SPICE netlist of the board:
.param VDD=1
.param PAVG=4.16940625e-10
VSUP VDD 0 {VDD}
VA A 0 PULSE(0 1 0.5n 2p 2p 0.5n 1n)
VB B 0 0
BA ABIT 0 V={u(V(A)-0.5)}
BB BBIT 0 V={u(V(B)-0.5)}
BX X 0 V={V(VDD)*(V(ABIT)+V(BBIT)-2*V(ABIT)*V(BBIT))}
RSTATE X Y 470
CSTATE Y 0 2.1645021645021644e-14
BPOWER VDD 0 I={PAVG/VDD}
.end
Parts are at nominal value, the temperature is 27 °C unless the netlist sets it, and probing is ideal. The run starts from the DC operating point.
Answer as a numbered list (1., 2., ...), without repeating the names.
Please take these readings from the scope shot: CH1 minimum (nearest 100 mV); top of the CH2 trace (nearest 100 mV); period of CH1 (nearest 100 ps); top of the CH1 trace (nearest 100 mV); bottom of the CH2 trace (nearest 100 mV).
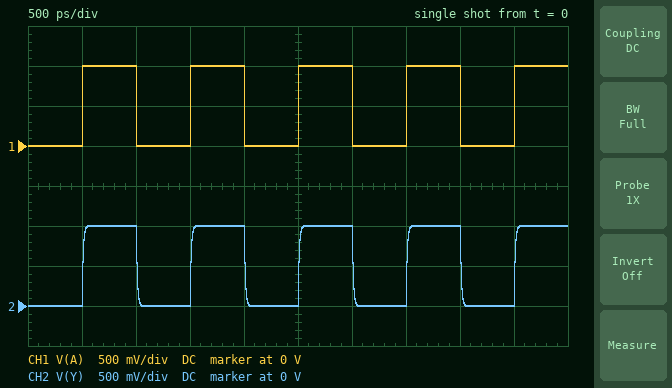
1. 0 V
2. 1.0 V
3. 1.0 ns
4. 1.0 V
5. 0 V
